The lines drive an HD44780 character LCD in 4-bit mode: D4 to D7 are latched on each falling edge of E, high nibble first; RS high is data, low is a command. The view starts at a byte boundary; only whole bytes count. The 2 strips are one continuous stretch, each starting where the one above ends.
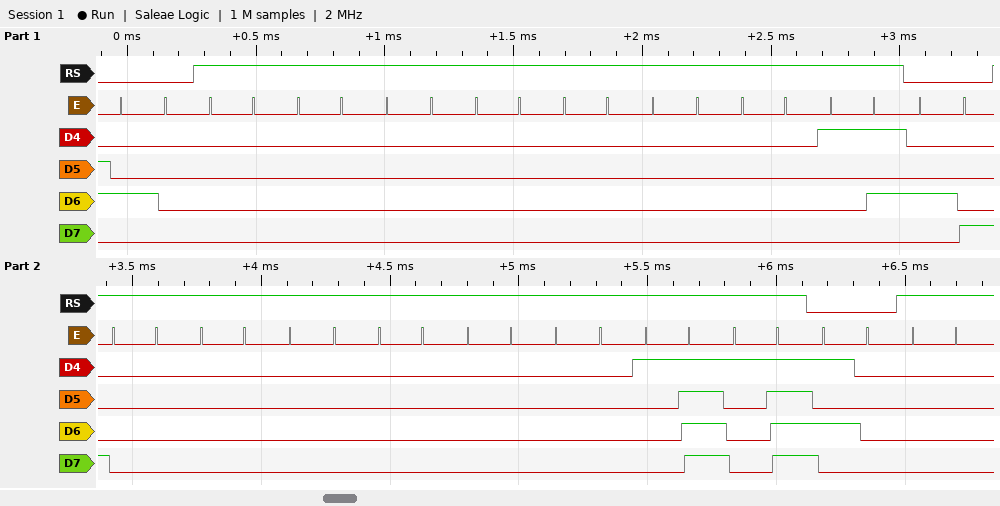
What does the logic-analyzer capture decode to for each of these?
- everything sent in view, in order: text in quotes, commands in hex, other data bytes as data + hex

0x40 data 00 00 00 00 00 00 00 15 0x48 data 00 00 00 00 00 00 1F 1F 0x50 data 00
